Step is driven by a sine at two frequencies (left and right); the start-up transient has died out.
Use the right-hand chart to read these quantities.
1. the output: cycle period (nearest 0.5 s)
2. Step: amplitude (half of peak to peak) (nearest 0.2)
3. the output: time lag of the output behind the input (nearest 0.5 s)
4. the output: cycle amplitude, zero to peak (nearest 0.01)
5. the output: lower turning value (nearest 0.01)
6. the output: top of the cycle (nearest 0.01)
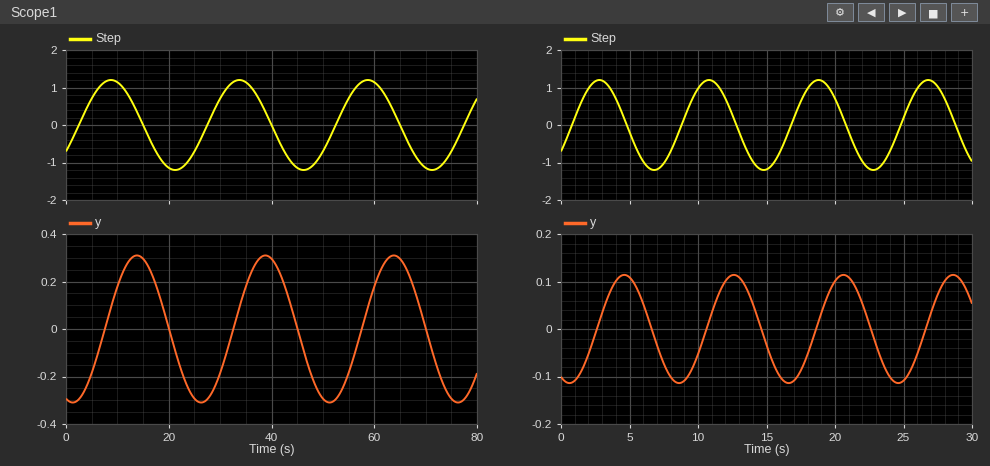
8.0 s
1.2
2.0 s
0.11
-0.11
0.11
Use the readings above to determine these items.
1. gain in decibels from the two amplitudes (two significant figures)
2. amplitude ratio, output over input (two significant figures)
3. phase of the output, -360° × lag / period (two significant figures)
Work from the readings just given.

-21 dB
0.092
-90°
